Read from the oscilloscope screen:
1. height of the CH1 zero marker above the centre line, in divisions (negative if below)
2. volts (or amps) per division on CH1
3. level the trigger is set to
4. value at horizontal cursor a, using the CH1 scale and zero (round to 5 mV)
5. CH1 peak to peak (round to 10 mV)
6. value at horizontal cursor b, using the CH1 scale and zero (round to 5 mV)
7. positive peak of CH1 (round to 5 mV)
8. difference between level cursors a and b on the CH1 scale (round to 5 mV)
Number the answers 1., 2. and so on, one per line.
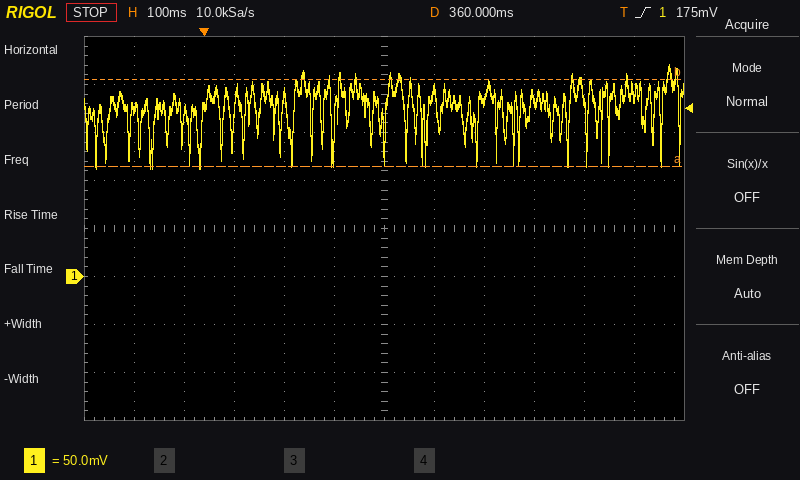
1. -1.0 div
2. 50 mV
3. 175 mV
4. 115 mV
5. 110 mV
6. 205 mV
7. 220 mV
8. 90 mV
